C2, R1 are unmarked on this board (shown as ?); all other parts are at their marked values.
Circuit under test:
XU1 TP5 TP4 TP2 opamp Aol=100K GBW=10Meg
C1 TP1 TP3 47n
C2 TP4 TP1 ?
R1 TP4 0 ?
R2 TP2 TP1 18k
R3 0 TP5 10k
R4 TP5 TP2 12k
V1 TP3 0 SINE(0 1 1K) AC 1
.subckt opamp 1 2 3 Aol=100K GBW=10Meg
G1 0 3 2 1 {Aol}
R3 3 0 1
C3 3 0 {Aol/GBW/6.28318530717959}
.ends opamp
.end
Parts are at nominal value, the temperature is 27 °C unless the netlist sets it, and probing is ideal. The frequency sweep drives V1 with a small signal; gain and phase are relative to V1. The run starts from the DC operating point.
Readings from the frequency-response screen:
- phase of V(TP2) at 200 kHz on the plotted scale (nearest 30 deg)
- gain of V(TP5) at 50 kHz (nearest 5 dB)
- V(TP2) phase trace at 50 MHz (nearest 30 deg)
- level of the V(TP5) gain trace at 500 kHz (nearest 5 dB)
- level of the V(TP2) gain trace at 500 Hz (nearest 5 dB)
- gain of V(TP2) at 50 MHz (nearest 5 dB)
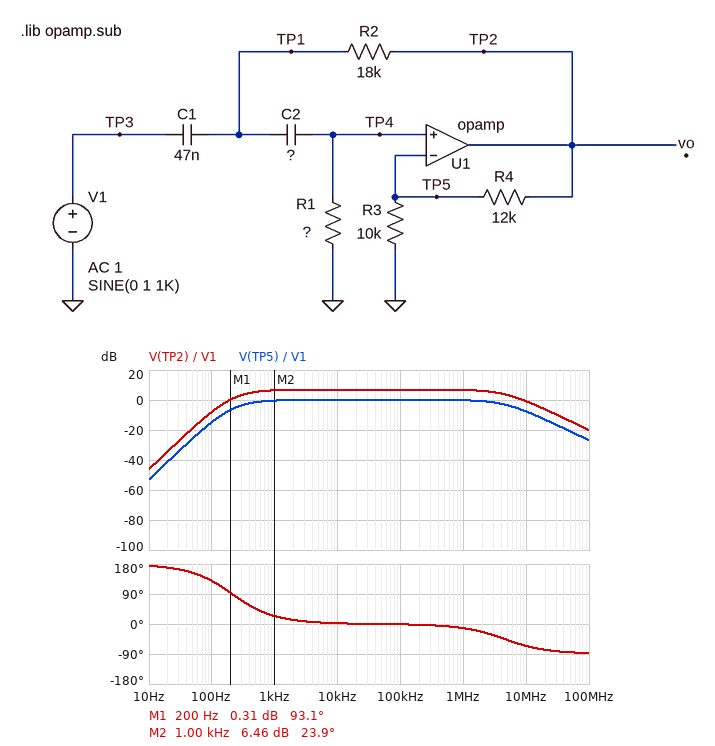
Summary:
0 deg
0 dB
-90 deg
0 dB
5 dB
-15 dB
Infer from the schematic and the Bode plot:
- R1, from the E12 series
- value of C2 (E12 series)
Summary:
8.2 kΩ
82 nF
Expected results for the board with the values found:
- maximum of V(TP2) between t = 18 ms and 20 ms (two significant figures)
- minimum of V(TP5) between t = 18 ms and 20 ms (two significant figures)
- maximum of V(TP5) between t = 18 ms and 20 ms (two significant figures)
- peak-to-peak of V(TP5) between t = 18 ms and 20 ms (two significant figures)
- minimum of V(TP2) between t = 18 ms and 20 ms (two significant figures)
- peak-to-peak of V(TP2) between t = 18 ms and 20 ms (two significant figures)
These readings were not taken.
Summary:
2.1 V
-960 mV
960 mV
1.9 V
-2.1 V
4.2 V
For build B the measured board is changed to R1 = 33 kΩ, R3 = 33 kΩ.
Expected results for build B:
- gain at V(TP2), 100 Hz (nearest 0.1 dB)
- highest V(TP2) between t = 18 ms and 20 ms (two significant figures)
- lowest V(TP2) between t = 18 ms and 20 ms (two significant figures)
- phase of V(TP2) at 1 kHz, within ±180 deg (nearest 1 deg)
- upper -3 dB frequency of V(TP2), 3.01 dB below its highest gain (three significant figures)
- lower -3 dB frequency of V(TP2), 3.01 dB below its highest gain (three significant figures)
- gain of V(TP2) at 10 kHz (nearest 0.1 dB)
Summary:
3.3 dB
1.4 V
-1.4 V
5 deg
3.73 MHz
88.8 Hz
2.7 dB
